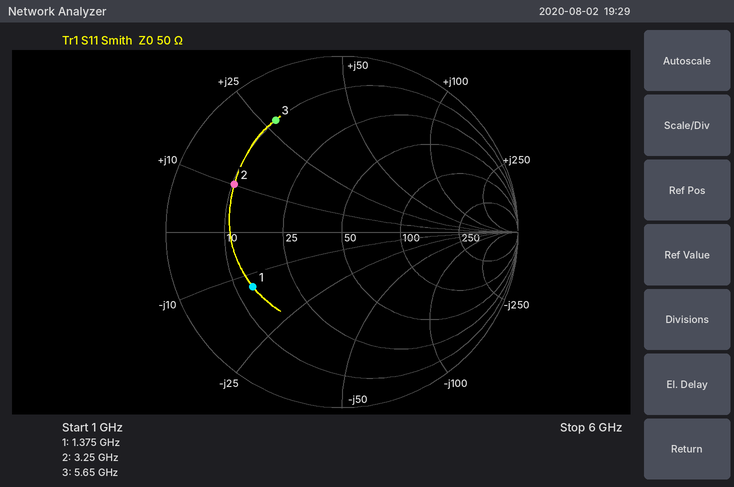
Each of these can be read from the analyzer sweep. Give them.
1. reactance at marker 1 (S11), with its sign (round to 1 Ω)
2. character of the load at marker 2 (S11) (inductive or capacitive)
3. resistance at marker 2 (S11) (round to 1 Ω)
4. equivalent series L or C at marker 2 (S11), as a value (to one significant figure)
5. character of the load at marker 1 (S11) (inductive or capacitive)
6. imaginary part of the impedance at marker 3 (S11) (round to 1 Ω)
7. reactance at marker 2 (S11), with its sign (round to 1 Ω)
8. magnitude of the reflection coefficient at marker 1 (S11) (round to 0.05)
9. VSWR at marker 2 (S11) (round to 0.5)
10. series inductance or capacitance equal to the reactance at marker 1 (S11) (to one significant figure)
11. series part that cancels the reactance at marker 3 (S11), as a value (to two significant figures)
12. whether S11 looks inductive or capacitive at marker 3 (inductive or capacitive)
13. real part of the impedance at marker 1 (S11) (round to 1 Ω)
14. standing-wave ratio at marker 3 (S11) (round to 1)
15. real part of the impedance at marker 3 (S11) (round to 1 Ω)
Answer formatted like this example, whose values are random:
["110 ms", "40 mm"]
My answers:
["-13 Ω", "inductive", "10 Ω", "500 pH", "capacitive", "+28 Ω", "+10 Ω", "0.60", "5.0", "9 pF", "1.0 pF", "inductive", "14 Ω", "7", "10 Ω"]
